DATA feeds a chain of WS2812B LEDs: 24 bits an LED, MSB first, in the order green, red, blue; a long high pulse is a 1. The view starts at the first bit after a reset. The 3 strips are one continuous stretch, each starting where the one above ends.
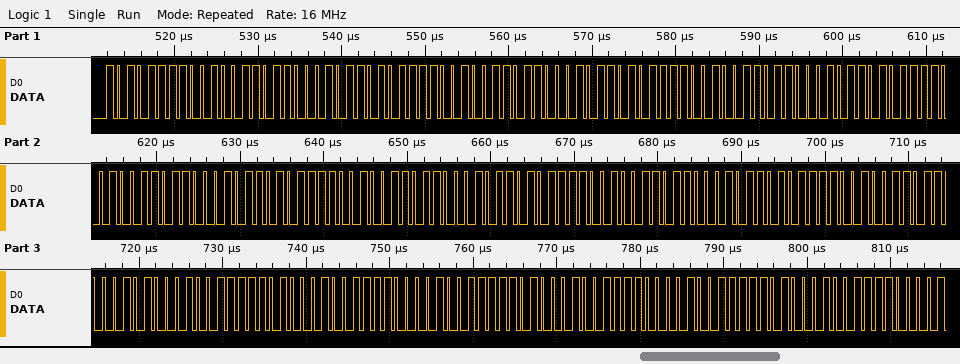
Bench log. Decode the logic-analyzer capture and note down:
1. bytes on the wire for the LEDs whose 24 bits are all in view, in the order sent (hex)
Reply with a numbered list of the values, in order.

1. AF 26 C5 AF 26 C5 AF 26 C5 AF 26 C5 AF 26 C5 AF 26 C5 AF 26 C5 13 E8 9E 13 E8 9E 13 E8 9E
